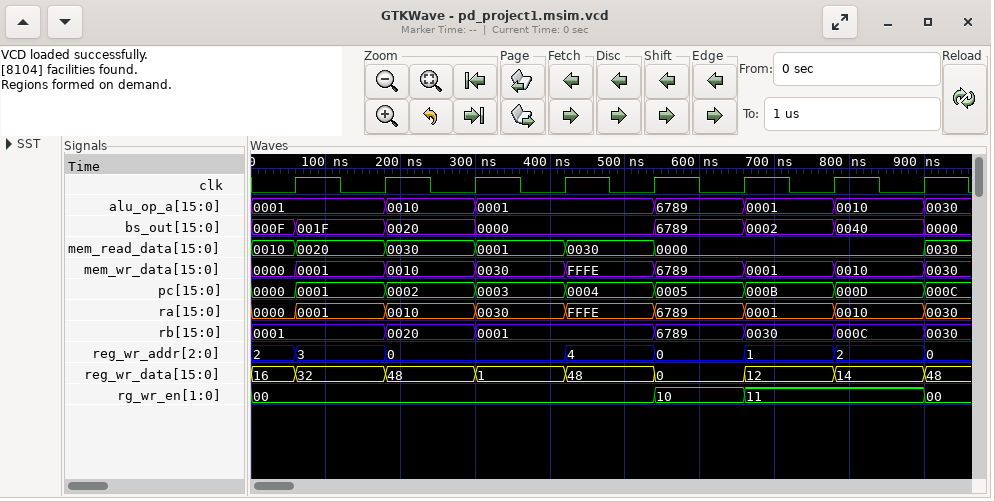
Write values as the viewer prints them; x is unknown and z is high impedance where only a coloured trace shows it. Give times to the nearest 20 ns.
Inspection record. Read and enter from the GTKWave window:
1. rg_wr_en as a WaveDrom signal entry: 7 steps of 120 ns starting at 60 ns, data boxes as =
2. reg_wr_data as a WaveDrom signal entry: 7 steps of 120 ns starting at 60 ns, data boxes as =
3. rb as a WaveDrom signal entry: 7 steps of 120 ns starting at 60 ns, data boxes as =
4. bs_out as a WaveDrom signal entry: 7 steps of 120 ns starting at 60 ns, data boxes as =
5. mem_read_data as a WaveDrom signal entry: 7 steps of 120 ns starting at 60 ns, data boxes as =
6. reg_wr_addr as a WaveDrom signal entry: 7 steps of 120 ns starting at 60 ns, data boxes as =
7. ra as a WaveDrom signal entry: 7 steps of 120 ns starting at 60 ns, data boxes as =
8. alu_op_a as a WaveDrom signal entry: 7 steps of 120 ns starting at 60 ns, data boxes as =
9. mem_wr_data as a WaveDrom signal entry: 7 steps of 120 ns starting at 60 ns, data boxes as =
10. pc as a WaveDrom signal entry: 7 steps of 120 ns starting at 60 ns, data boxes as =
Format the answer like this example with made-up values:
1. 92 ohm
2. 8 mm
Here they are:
1. {name: 'rg_wr_en', wave: '=...==.', data: '00 10 11'}
2. {name: 'reg_wr_data', wave: '=======', data: '32 48 1 48 0 12 14'}
3. {name: 'rb', wave: '===.===', data: '0001 0020 0001 6789 0030 000C'}
4. {name: 'bs_out', wave: '===.===', data: '001F 0020 0000 6789 0002 0040'}
5. {name: 'mem_read_data', wave: '=====..', data: '0020 0030 0001 0030 0000'}
6. {name: 'reg_wr_addr', wave: '==.====', data: '3 0 4 0 1 2'}
7. {name: 'ra', wave: '=======', data: '0001 0010 0030 FFFE 6789 0001 0010'}
8. {name: 'alu_op_a', wave: '===.===', data: '0001 0010 0001 6789 0001 0010'}
9. {name: 'mem_wr_data', wave: '=======', data: '0001 0010 0030 FFFE 6789 0001 0010'}
10. {name: 'pc', wave: '=======', data: '0001 0002 0003 0004 0005 000B 000D'}
